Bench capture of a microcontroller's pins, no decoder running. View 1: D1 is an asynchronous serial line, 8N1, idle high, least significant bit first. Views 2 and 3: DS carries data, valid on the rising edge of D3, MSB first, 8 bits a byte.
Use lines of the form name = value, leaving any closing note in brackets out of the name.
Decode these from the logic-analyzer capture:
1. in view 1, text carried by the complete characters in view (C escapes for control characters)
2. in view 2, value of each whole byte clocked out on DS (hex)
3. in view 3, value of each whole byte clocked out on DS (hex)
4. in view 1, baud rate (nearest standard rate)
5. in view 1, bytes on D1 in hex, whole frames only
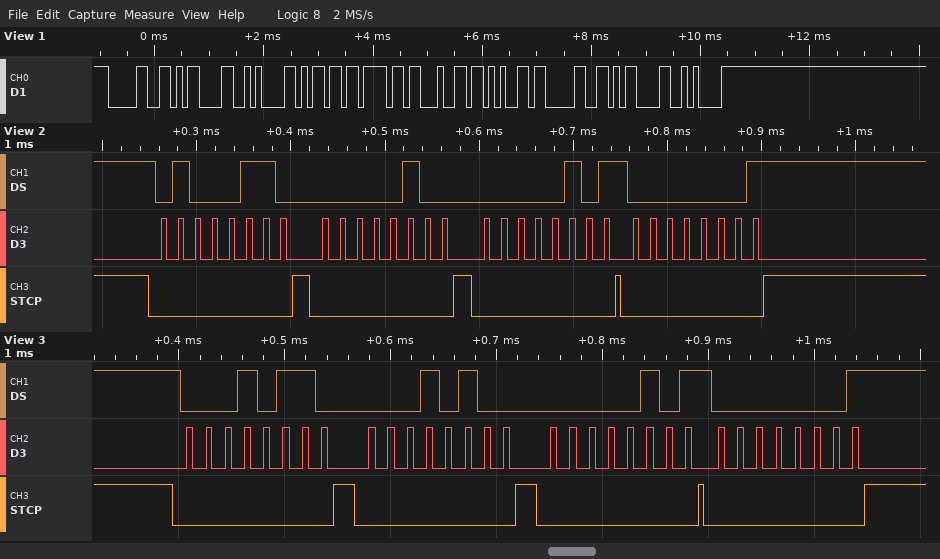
in view 1, text carried by the complete characters in view = "0\r\nmode0\r\n"
in view 2, value of each whole byte clocked out on DS = 46 04 05 01
in view 3, value of each whole byte clocked out on DS = 16 14 05 01
in view 1, baud rate = 9600 baud
in view 1, bytes on D1 in hex, whole frames only = 30 0D 0A 6D 6F 64 65 30 0D 0A
